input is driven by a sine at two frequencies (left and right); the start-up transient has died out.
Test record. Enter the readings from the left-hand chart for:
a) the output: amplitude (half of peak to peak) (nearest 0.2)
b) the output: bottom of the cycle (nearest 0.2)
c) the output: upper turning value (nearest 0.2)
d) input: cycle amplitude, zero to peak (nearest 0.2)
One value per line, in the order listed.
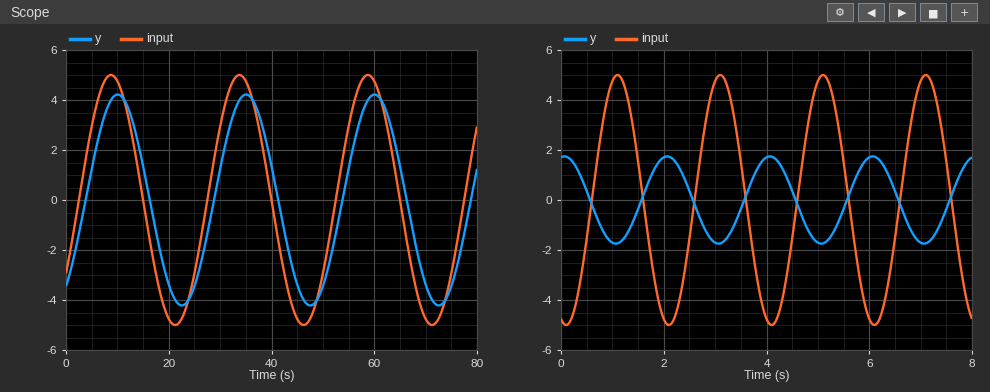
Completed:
4.2
-4.2
4.2
5.0
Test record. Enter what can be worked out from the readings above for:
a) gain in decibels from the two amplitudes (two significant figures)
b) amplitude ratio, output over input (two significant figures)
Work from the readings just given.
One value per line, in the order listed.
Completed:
-1.5 dB
0.84
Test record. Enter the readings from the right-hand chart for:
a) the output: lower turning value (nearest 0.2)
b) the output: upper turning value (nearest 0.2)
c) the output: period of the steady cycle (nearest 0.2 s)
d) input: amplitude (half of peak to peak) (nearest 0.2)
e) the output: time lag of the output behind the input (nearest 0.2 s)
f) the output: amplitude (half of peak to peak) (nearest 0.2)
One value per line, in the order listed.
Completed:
-1.8
1.8
2.0 s
5.0
1.0 s
1.8
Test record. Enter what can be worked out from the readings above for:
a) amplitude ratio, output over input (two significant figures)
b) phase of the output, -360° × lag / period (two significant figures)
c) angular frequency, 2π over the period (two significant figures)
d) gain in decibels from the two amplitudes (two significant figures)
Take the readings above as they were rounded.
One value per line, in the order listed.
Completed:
0.36
-180°
3.1 rad/s
-8.9 dB
